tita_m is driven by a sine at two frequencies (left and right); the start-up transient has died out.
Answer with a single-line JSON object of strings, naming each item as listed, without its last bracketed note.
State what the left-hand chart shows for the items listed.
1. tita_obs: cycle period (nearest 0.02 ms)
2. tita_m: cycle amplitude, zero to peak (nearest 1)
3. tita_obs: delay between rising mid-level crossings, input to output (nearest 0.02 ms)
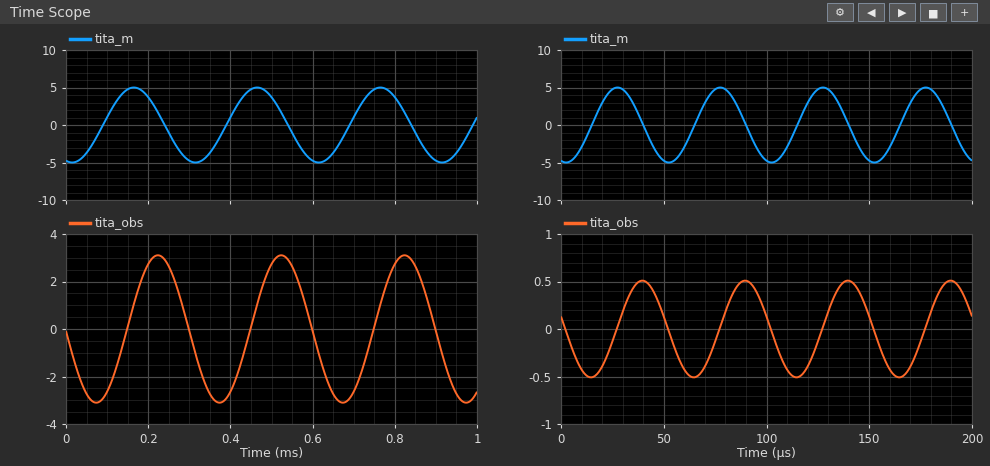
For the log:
{"tita_obs: cycle period": "0.30 ms", "tita_m: cycle amplitude, zero to peak": "5", "tita_obs: delay between rising mid-level crossings, input to output": "0.06 ms"}
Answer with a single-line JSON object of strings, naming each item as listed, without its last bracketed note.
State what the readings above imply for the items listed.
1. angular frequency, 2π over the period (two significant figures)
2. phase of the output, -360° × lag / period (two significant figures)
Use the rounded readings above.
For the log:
{"angular frequency, 2π over the period": "21 rad/ms", "phase of the output, -360° × lag / period": "-72°"}
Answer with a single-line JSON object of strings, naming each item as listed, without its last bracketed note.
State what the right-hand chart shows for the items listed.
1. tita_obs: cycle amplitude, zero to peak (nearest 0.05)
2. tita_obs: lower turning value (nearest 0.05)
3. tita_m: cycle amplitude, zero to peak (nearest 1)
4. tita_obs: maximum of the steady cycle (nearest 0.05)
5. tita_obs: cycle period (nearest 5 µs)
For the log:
{"tita_obs: cycle amplitude, zero to peak": "0.50", "tita_obs: lower turning value": "-0.50", "tita_m: cycle amplitude, zero to peak": "5", "tita_obs: maximum of the steady cycle": "0.50", "tita_obs: cycle period": "50 µs"}
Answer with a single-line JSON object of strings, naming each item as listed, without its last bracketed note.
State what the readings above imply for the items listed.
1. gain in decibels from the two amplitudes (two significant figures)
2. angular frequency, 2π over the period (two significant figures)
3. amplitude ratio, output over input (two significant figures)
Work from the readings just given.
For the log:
{"gain in decibels from the two amplitudes": "-20 dB", "angular frequency, 2π over the period": "0.13 rad/µs", "amplitude ratio, output over input": "0.10"}
